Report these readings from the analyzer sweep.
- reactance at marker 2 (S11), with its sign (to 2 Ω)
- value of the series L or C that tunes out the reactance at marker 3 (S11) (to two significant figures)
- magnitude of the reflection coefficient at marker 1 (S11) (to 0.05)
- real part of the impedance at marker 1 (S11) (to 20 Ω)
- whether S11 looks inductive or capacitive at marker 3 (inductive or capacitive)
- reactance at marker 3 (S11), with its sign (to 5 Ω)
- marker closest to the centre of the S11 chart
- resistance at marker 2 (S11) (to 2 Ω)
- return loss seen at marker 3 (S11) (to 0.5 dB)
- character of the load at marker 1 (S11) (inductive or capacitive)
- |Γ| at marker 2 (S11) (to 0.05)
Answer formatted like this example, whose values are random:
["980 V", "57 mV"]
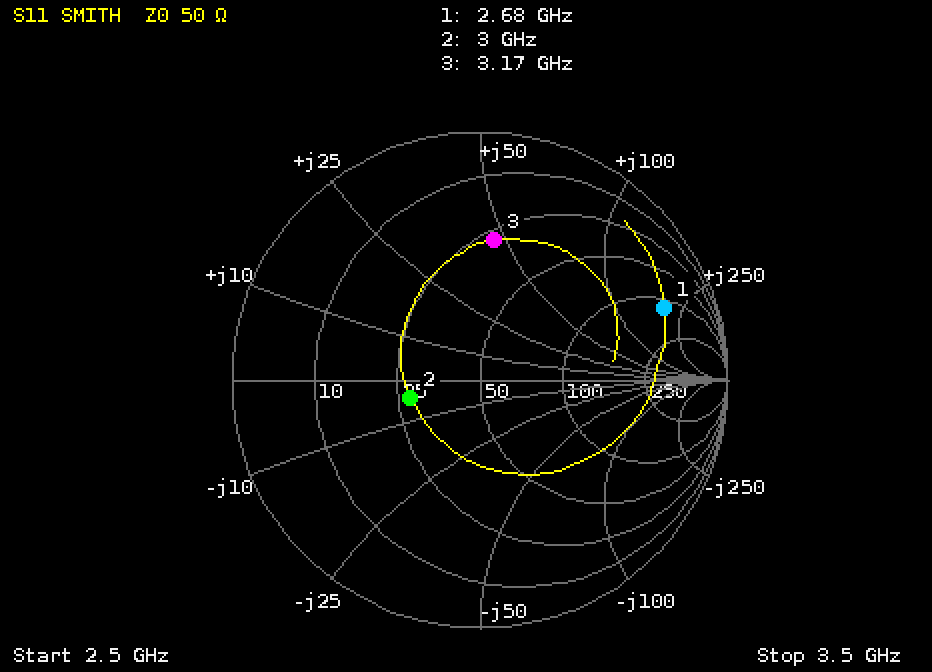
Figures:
["-4 Ω", "1.1 pF", "0.80", "120 Ω", "inductive", "+45 Ω", "marker 2", "28 Ω", "5.0 dB", "inductive", "0.30"]
